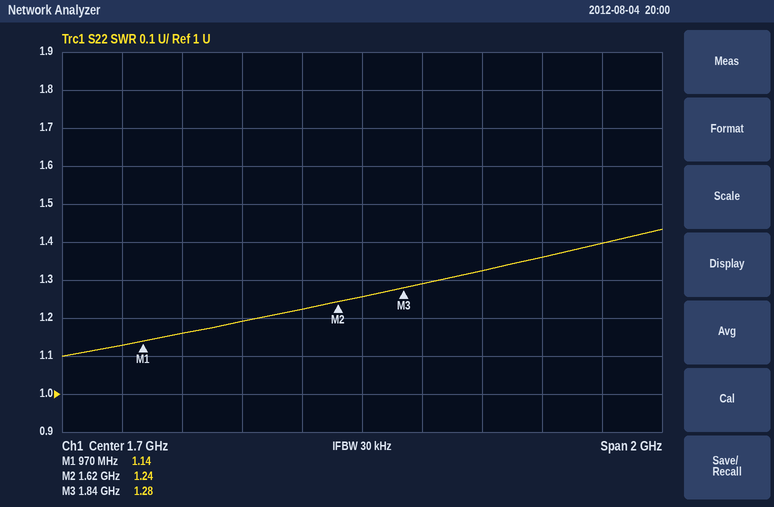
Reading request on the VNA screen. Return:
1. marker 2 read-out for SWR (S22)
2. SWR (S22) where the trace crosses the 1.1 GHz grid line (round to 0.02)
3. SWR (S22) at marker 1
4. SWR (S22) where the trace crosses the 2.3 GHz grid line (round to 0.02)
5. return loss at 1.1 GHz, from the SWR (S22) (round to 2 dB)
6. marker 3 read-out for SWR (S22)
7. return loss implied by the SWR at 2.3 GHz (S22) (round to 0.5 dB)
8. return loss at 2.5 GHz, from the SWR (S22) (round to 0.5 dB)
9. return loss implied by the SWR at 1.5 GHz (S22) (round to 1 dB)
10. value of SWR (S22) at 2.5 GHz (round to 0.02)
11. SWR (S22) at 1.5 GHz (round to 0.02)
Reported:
1.24
1.16
1.14
1.36
22 dB
1.28
16.5 dB
15.5 dB
20 dB
1.40
1.22
